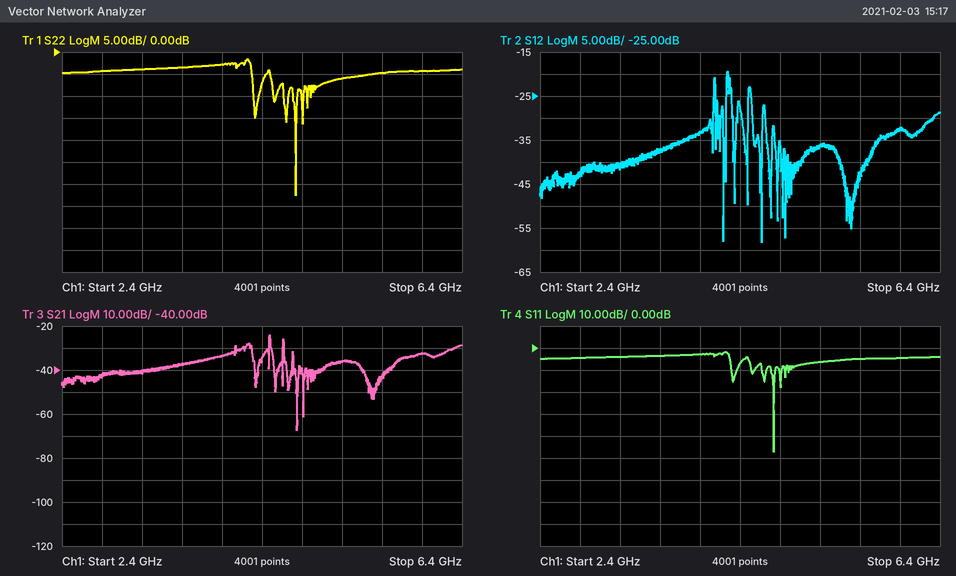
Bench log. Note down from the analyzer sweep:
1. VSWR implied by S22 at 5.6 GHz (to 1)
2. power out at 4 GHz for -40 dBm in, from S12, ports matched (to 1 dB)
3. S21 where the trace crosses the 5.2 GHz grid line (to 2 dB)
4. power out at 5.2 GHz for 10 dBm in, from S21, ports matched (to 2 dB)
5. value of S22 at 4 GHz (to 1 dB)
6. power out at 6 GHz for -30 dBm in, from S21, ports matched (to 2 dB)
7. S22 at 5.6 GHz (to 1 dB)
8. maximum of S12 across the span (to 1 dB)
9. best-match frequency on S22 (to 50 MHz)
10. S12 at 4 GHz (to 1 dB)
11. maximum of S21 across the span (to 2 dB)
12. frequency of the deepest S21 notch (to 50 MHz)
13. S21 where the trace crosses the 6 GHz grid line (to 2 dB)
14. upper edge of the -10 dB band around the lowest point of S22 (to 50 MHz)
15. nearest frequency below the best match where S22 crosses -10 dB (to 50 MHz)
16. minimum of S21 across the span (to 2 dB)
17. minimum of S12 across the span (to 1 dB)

4
-73 dBm
-36 dB
-26 dBm
-3 dB
-62 dBm
-5 dB
-19 dB
4.75 GHz
-33 dB
-24 dB
4.75 GHz
-32 dB
4.75 GHz
4.70 GHz
-68 dB
-58 dB
